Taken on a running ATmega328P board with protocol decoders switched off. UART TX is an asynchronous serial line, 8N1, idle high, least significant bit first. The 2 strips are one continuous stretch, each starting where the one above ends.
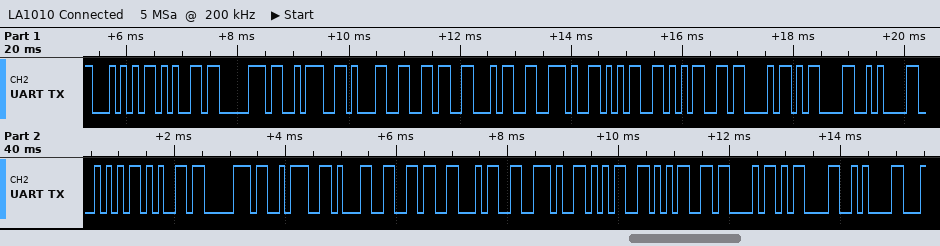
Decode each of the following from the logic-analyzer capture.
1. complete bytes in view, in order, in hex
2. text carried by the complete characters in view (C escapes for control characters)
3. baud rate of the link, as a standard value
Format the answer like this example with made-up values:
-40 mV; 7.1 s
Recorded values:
54 65 70 3A 31 36 34 2E 35 35 43 0D 0A 54 65 70 3A 31 36 34 2E 35 35 43 0D 0A; "Tep:164.55C\r\nTep:164.55C\r\n"; 9600 baud
